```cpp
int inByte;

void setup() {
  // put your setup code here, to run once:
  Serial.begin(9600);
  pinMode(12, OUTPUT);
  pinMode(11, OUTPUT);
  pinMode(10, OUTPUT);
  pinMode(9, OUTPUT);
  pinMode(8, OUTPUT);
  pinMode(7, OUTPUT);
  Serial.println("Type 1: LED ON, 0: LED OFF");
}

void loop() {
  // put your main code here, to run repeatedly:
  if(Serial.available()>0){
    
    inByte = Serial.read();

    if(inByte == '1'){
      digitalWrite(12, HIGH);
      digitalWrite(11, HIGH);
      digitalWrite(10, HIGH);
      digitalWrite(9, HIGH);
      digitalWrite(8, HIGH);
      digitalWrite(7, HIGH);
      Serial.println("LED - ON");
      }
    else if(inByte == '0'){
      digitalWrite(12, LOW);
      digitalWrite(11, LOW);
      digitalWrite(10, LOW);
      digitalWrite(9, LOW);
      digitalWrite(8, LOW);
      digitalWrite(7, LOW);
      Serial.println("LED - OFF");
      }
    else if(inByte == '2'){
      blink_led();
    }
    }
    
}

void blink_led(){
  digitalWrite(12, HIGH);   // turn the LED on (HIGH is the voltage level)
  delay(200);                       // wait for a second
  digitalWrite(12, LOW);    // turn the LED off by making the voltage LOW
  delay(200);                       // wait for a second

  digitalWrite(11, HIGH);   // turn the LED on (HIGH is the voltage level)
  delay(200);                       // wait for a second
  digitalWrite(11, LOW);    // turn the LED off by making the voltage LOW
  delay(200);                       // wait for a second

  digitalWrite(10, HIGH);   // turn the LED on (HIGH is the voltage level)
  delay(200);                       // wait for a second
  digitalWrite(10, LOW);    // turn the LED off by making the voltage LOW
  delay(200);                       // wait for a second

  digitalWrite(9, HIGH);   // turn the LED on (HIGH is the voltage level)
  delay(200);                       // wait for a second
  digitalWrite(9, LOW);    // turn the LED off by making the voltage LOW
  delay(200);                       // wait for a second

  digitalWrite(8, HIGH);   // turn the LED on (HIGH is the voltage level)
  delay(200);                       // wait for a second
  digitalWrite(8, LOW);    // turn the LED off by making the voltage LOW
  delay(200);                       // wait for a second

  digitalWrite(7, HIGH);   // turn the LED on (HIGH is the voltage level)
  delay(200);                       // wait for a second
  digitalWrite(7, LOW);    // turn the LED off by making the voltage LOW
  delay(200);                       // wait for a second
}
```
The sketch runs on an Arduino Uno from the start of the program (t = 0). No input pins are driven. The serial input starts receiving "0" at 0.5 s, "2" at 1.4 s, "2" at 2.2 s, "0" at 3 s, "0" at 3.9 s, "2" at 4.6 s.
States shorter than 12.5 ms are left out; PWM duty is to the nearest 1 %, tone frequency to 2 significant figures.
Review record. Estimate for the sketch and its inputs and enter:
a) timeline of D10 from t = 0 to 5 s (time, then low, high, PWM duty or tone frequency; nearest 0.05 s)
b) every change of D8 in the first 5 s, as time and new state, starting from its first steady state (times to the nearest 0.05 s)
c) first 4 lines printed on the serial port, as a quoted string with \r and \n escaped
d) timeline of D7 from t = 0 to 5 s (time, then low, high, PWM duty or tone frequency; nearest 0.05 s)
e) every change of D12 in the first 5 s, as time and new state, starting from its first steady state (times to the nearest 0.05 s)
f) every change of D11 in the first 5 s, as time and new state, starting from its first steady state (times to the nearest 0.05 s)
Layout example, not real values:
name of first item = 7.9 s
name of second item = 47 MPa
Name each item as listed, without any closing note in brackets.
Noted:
timeline of D10 from t = 0 to 5 s = 0 s low; 2.2 s high; 2.4 s low; 4.6 s high; 4.8 s low
every change of D8 in the first 5 s, as time and new state, starting from its first steady state = 0 s low; 3 s high; 3.2 s low
first 4 lines printed on the serial port, as a quoted string with \r and \n escaped = "Type 1: LED ON, 0: LED OFF\r\nLED - OFF\r\nLED - OFF\r\nLED - OFF\r\n"
timeline of D7 from t = 0 to 5 s = 0 s low; 3.4 s high; 3.6 s low
every change of D12 in the first 5 s, as time and new state, starting from its first steady state = 0 s low; 1.4 s high; 1.6 s low; 3.8 s high; 4 s low
every change of D11 in the first 5 s, as time and new state, starting from its first steady state = 0 s low; 1.8 s high; 2 s low; 4.2 s high; 4.4 s low
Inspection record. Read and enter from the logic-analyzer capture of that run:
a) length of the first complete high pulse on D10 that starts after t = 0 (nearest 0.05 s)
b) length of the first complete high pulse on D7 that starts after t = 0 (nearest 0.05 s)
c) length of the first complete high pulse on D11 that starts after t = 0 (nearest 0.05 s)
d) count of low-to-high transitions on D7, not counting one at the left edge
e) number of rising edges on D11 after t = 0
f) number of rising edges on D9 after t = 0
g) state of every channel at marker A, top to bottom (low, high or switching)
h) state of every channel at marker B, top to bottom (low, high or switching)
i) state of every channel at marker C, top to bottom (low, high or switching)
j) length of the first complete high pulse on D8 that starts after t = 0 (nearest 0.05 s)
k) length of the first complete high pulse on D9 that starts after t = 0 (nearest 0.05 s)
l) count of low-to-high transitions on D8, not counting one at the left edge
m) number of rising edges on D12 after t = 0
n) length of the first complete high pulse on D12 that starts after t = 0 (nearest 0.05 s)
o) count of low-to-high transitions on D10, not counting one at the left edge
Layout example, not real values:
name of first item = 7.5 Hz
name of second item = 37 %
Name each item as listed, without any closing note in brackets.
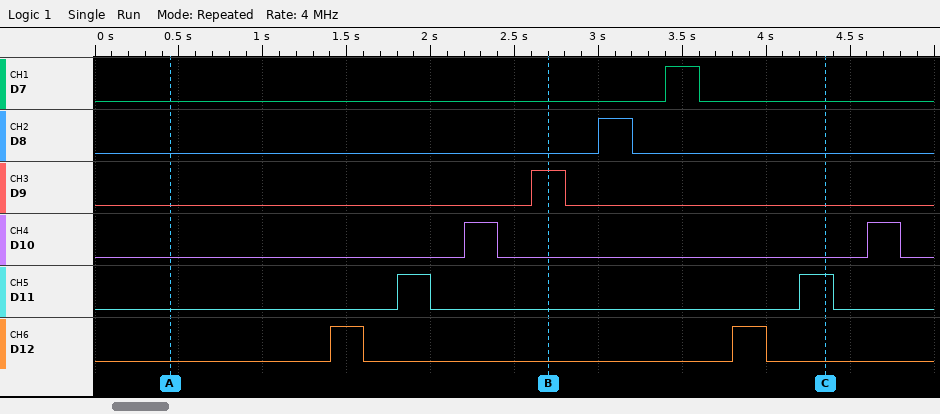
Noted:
length of the first complete high pulse on D10 that starts after t = 0 = 0.20 s
length of the first complete high pulse on D7 that starts after t = 0 = 0.20 s
length of the first complete high pulse on D11 that starts after t = 0 = 0.20 s
count of low-to-high transitions on D7, not counting one at the left edge = 1
number of rising edges on D11 after t = 0 = 2
number of rising edges on D9 after t = 0 = 1
state of every channel at marker A, top to bottom = D7 low, D8 low, D9 low, D10 low, D11 low, D12 low
state of every channel at marker B, top to bottom = D7 low, D8 low, D9 high, D10 low, D11 low, D12 low
state of every channel at marker C, top to bottom = D7 low, D8 low, D9 low, D10 low, D11 high, D12 low
length of the first complete high pulse on D8 that starts after t = 0 = 0.20 s
length of the first complete high pulse on D9 that starts after t = 0 = 0.20 s
count of low-to-high transitions on D8, not counting one at the left edge = 1
number of rising edges on D12 after t = 0 = 2
length of the first complete high pulse on D12 that starts after t = 0 = 0.20 s
count of low-to-high transitions on D10, not counting one at the left edge = 2
